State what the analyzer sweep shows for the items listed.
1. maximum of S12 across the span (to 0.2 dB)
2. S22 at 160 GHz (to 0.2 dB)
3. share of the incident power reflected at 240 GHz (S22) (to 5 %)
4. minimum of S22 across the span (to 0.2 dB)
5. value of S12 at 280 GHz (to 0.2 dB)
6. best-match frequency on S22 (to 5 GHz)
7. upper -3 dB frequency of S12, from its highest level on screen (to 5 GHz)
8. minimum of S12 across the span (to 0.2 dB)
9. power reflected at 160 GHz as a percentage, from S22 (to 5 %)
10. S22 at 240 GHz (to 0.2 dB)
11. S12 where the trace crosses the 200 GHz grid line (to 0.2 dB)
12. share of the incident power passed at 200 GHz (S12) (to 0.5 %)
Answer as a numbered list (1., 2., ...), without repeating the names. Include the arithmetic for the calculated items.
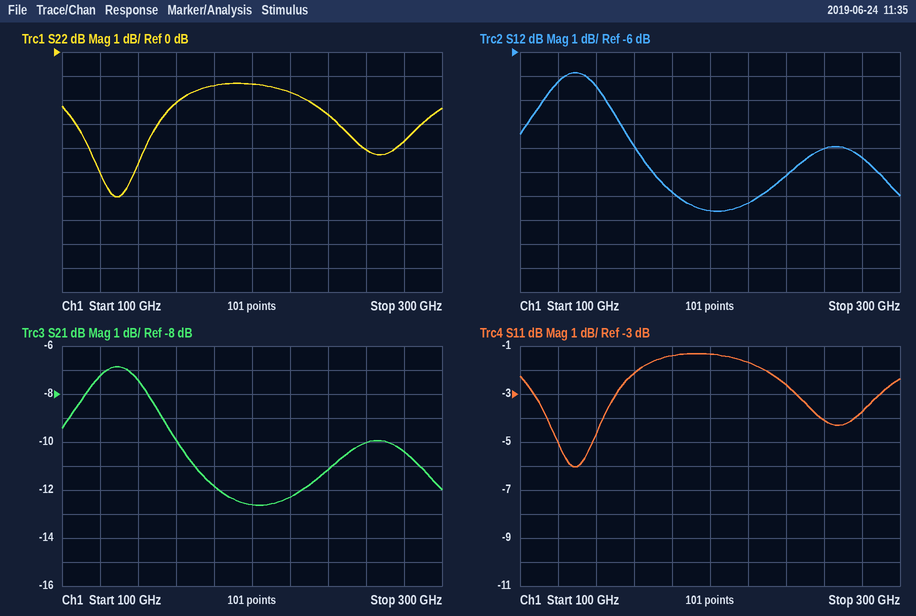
1. -6.8 dB
2. -2.2 dB
3. 10^(-2.6/10) ≈ 55 %
4. -6.0 dB
5. -10.4 dB
6. 130 GHz
7. 160 GHz
8. -12.6 dB
9. 10^(-2.2/10) ≈ 60 %
10. -2.6 dB
11. -12.6 dB
12. 10^(-12.6/10) ≈ 5.5 %
